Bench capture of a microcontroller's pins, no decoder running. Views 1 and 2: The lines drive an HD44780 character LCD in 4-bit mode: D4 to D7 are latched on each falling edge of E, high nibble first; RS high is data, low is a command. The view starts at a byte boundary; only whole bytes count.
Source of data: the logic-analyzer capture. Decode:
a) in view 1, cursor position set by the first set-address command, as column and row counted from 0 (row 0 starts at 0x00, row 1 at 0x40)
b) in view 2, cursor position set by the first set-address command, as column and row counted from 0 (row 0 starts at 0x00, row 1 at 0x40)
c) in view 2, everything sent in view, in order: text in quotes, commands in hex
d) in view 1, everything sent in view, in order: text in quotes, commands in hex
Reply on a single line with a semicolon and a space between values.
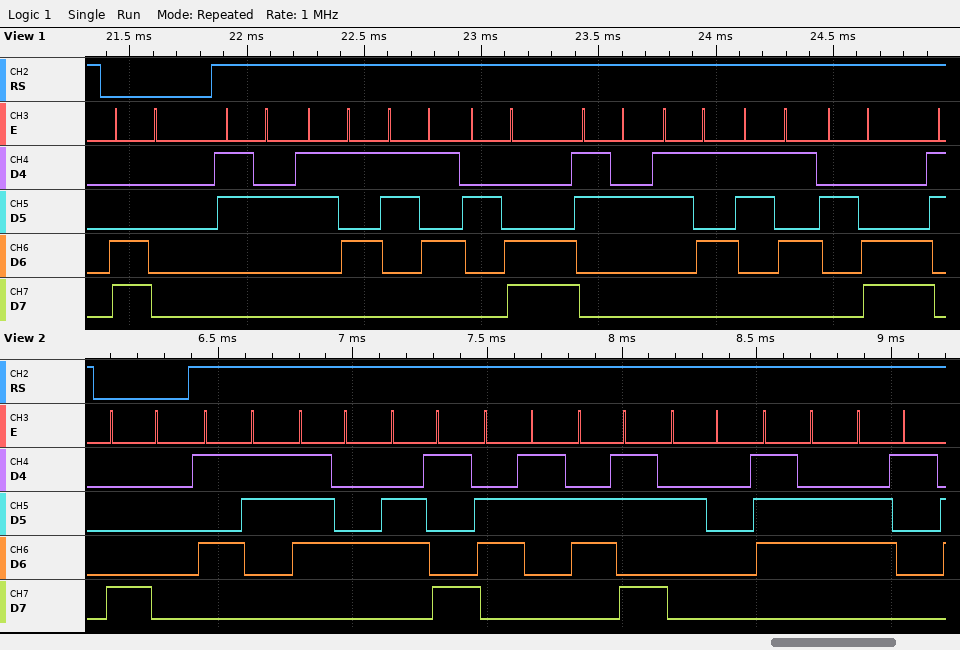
column 0, row 1; column 0, row 0; 0x80 "Stick va"; 0xC0 "255,255,"
